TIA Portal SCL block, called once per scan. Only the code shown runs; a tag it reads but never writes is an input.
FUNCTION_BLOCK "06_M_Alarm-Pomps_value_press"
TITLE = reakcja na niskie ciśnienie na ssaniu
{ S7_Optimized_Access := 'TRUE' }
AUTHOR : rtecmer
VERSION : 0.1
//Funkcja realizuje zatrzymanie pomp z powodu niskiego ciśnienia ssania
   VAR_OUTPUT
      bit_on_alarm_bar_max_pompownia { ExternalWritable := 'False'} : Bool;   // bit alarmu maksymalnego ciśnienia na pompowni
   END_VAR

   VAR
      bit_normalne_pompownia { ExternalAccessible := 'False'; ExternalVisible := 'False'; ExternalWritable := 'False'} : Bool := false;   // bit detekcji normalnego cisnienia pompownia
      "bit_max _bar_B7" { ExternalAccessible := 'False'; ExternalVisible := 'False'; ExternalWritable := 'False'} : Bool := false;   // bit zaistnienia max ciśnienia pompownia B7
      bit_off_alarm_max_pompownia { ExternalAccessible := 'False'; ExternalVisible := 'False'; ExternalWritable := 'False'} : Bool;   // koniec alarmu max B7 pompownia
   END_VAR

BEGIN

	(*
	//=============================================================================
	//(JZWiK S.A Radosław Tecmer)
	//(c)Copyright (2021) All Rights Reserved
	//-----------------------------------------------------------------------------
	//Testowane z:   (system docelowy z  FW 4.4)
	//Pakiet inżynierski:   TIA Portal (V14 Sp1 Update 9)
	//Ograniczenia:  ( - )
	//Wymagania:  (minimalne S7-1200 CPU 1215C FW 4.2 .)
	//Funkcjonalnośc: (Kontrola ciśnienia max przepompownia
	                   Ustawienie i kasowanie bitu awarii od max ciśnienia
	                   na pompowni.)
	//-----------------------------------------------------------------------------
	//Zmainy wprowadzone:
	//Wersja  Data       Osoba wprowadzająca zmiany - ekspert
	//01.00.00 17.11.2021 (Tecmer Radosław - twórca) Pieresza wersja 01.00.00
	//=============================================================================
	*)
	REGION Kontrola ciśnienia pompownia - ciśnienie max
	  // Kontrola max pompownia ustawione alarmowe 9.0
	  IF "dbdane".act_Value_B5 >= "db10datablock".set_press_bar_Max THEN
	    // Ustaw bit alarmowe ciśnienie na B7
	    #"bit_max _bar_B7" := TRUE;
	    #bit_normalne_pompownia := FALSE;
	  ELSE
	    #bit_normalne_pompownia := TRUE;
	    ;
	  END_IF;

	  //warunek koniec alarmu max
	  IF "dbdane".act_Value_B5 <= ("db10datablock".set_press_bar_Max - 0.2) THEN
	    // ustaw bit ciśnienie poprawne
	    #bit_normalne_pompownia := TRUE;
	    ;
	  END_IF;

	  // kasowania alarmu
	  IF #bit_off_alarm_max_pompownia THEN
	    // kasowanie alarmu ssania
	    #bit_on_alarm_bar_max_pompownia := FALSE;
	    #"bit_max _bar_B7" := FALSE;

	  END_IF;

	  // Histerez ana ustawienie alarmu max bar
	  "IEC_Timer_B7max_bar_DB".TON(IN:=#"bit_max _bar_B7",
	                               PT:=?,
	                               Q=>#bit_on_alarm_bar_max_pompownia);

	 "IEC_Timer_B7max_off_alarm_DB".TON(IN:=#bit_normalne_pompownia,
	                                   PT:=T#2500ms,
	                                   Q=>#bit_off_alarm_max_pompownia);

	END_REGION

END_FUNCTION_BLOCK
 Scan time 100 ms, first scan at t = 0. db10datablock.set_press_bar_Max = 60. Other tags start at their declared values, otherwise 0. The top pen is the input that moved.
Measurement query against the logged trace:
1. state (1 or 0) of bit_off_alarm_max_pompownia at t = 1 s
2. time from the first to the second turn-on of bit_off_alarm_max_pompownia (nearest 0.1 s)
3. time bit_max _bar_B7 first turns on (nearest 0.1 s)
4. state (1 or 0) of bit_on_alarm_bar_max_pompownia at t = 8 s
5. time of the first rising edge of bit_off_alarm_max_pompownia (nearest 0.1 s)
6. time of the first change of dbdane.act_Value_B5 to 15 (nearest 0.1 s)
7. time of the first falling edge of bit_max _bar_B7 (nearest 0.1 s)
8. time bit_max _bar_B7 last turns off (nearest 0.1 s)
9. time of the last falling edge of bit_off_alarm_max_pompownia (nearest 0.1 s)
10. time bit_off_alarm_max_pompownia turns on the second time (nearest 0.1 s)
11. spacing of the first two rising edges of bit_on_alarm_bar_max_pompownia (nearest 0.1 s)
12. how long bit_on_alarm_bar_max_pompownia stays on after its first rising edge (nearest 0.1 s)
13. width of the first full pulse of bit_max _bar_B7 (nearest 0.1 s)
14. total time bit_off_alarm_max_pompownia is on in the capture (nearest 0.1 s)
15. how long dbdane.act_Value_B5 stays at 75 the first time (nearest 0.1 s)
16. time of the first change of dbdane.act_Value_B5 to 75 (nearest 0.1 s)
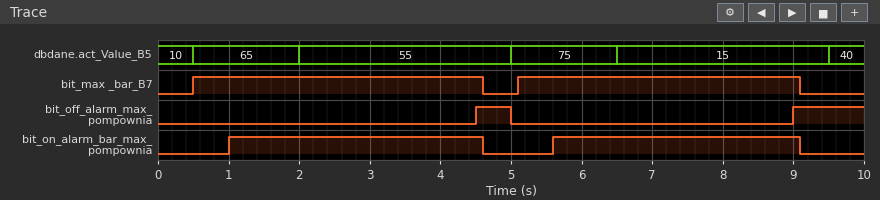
0
4.5 s
0.5 s
1
4.5 s
6.5 s
4.6 s
9.1 s
5.0 s
9.0 s
4.6 s
3.6 s
4.1 s
1.5 s
1.5 s
5.0 s
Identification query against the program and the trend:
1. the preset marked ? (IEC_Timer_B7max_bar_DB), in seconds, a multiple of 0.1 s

0.5 s
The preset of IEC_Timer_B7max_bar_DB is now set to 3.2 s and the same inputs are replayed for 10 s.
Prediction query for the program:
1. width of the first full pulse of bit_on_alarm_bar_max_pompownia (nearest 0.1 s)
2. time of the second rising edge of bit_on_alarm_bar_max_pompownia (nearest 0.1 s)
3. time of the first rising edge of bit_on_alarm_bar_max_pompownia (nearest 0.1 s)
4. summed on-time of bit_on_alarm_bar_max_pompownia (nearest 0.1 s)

0.9 s
8.3 s
3.7 s
1.7 s
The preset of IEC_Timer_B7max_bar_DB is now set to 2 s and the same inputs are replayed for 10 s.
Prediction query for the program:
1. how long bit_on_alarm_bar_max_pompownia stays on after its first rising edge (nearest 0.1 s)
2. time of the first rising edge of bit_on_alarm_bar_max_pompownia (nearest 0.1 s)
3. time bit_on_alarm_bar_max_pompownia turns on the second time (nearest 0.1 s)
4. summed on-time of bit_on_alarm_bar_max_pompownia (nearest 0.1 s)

2.1 s
2.5 s
7.1 s
4.1 s
